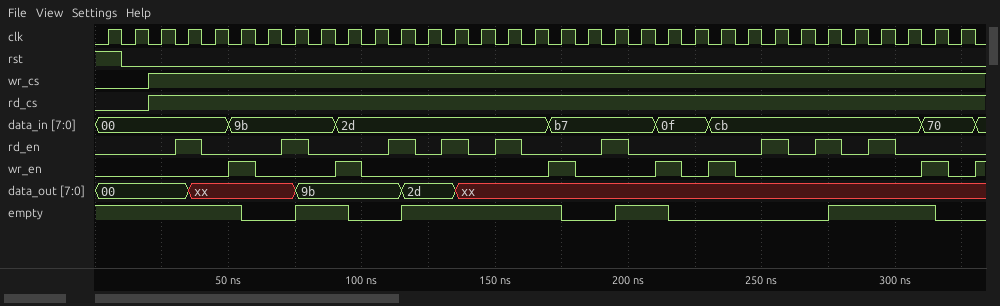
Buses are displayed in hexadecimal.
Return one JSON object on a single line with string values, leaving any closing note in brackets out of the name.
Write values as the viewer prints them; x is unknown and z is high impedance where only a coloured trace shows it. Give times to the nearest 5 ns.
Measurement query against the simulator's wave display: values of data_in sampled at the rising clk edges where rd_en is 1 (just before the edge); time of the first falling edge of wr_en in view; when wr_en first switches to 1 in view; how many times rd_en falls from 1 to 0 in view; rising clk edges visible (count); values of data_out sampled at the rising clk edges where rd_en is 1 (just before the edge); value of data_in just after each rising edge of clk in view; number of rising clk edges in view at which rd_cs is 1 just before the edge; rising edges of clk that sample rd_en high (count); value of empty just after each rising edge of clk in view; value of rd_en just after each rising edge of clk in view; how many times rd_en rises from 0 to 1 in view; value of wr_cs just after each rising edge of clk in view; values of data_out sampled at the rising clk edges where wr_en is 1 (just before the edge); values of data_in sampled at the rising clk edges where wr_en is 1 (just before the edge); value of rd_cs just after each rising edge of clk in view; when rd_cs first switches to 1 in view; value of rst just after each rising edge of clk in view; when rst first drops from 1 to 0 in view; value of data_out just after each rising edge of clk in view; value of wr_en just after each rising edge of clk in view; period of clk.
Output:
{"values of data_in sampled at the rising clk edges where rd_en is 1": "00, 9b, 2d, 2d, 2d, b7, cb, cb, cb", "time of the first falling edge of wr_en in view": "60 ns", "when wr_en first switches to 1 in view": "50 ns", "how many times rd_en falls from 1 to 0 in view": "9", "rising clk edges visible": "33", "values of data_out sampled at the rising clk edges where rd_en is 1": "00, xx, 9b, 2d, xx, xx, xx, xx, xx", "value of data_in just after each rising edge of clk in view": "00, 00, 00, 00, 00, 9b, 9b, 9b, 9b, 2d, 2d, 2d, 2d, 2d, 2d, 2d, 2d, b7, b7, b7, b7, 0f, 0f, cb, cb, cb, cb, cb, cb, cb, cb, 70, 70", "number of rising clk edges in view at which rd_cs is 1 just before the edge": "31", "rising edges of clk that sample rd_en high": "9", "value of empty just after each rising edge of clk in view": "1 1 1 1 1 0 0 1 1 0 0 1 1 1 1 1 1 0 0 1 1 0 0 0 0 0 0 1 1 1 1 0 0", "value of rd_en just after each rising edge of clk in view": "0 0 0 1 0 0 0 1 0 0 0 1 0 1 0 1 0 0 0 1 0 0 0 0 0 1 0 1 0 1 0 0 0", "how many times rd_en rises from 0 to 1 in view": "9", "value of wr_cs just after each rising edge of clk in view": "0 0 1 1 1 1 1 1 1 1 1 1 1 1 1 1 1 1 1 1 1 1 1 1 1 1 1 1 1 1 1 1 1", "values of data_out sampled at the rising clk edges where wr_en is 1": "xx, 9b, xx, xx, xx, xx", "values of data_in sampled at the rising clk edges where wr_en is 1": "9b, 2d, b7, 0f, cb, 70", "value of rd_cs just after each rising edge of clk in view": "0 0 1 1 1 1 1 1 1 1 1 1 1 1 1 1 1 1 1 1 1 1 1 1 1 1 1 1 1 1 1 1 1", "when rd_cs first switches to 1 in view": "20 ns", "value of rst just after each rising edge of clk in view": "1 0 0 0 0 0 0 0 0 0 0 0 0 0 0 0 0 0 0 0 0 0 0 0 0 0 0 0 0 0 0 0 0", "when rst first drops from 1 to 0 in view": "10 ns", "value of data_out just after each rising edge of clk in view": "00, 00, 00, xx, xx, xx, xx, 9b, 9b, 9b, 9b, 2d, 2d, xx, xx, xx, xx, xx, xx, xx, xx, xx, xx, xx, xx, xx, xx, xx, xx, xx, xx, xx, xx", "value of wr_en just after each rising edge of clk in view": "0 0 0 0 0 1 0 0 0 1 0 0 0 0 0 0 0 1 0 0 0 1 0 1 0 0 0 0 0 0 0 1 0", "period of clk": "10 ns"}
